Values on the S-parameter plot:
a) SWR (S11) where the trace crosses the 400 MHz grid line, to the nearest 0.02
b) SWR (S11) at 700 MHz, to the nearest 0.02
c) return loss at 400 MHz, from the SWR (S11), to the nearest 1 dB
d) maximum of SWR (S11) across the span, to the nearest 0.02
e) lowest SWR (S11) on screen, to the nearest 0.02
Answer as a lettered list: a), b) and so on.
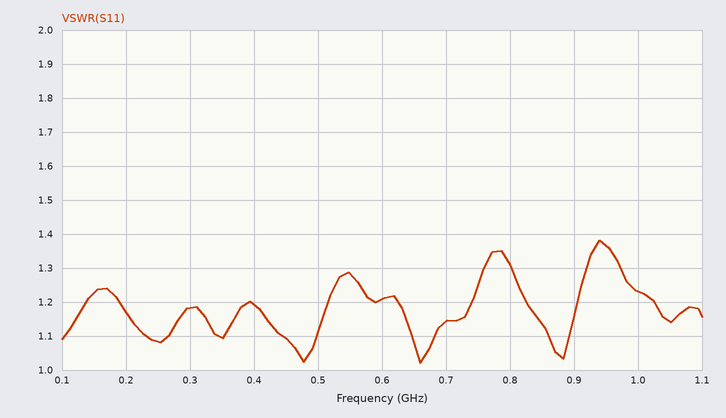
a) 1.20
b) 1.14
c) 21 dB
d) 1.38
e) 1.02
